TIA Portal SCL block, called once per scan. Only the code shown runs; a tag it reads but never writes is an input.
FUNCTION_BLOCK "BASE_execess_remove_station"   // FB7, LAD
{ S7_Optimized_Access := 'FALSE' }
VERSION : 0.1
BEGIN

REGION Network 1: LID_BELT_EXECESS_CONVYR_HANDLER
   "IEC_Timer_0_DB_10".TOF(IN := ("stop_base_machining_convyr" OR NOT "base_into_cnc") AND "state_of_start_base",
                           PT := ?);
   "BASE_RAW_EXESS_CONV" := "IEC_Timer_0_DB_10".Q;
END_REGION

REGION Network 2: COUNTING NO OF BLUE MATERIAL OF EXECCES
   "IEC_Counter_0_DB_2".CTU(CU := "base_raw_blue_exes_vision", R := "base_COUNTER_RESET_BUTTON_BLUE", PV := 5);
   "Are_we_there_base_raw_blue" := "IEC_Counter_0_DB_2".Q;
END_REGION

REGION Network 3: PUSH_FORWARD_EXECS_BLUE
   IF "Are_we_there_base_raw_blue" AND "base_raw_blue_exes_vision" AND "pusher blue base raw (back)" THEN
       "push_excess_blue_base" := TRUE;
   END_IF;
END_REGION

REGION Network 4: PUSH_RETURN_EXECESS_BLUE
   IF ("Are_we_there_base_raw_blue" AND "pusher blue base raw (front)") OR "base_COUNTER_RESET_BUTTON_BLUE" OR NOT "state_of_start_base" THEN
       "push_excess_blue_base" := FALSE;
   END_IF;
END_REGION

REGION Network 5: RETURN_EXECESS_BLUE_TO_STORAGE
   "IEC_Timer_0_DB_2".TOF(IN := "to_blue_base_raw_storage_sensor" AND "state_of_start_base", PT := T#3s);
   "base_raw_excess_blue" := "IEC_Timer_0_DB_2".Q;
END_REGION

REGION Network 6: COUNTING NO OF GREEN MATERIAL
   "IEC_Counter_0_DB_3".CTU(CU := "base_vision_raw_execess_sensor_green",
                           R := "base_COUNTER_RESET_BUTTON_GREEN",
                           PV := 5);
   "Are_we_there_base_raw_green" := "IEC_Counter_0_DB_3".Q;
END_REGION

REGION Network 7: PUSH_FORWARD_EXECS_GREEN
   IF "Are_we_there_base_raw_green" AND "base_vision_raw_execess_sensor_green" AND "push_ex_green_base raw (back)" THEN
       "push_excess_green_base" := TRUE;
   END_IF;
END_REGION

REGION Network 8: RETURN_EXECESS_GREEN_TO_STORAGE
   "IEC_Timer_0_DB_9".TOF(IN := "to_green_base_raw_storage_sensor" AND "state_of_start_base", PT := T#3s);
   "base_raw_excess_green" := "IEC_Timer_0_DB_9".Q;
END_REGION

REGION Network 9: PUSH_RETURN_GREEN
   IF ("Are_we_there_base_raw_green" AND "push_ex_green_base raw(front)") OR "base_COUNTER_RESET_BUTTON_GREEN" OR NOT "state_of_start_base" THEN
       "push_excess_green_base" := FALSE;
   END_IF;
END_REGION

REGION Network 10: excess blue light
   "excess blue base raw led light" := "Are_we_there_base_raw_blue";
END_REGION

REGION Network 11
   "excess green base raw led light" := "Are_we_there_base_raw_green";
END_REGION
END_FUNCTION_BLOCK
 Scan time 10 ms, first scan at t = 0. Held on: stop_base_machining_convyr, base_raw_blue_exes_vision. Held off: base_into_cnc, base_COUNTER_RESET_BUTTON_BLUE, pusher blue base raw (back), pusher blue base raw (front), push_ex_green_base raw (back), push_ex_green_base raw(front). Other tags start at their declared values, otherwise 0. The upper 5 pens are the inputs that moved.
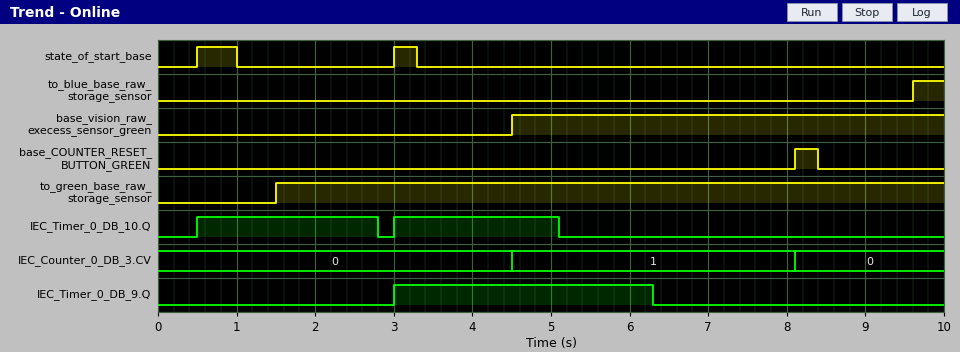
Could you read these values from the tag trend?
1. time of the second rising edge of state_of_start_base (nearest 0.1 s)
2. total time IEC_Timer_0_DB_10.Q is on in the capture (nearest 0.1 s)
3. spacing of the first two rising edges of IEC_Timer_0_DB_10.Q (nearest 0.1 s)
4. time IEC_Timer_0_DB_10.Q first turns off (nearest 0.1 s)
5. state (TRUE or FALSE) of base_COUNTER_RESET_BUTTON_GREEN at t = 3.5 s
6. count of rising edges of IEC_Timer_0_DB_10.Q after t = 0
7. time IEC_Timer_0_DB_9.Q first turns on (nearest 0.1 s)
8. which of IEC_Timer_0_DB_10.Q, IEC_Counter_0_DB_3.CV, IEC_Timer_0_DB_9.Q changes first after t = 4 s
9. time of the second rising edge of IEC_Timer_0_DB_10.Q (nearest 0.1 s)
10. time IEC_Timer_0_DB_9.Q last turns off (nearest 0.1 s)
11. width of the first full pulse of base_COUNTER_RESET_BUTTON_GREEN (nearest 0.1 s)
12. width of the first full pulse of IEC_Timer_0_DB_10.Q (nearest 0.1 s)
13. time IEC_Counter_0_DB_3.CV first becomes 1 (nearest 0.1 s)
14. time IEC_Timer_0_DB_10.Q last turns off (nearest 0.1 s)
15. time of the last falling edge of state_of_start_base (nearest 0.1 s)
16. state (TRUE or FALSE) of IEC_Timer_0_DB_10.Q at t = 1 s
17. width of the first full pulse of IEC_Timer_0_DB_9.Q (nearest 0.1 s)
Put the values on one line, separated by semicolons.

3.0 s; 4.4 s; 2.5 s; 2.8 s; FALSE; 2; 3.0 s; IEC_Counter_0_DB_3.CV; 3.0 s; 6.3 s; 0.3 s; 2.3 s; 4.5 s; 5.1 s; 3.3 s; TRUE; 3.3 s
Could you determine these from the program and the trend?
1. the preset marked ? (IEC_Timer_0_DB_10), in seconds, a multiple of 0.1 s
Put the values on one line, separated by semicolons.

1.8 s
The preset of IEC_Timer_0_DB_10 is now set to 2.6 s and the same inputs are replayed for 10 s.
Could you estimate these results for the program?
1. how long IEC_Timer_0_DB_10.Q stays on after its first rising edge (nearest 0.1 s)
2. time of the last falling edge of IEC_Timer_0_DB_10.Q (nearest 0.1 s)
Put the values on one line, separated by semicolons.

5.4 s; 5.9 s
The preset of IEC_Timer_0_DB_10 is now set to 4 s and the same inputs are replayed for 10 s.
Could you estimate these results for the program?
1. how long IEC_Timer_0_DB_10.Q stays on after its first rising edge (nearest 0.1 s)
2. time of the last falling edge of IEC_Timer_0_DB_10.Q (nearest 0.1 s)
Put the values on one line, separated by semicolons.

6.8 s; 7.3 s
